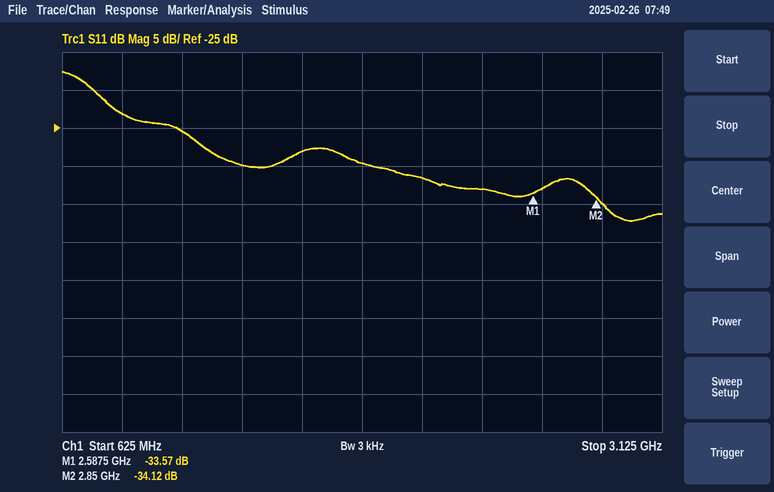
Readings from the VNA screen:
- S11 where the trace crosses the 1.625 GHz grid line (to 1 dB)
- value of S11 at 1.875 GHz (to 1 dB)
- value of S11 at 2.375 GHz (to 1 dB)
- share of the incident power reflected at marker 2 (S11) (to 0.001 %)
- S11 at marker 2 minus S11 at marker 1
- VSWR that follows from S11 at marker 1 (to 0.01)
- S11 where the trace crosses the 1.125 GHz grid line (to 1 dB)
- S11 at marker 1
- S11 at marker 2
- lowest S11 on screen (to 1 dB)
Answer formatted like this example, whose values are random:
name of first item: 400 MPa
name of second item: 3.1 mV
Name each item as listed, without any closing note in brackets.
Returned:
S11 where the trace crosses the 1.625 GHz grid line: -28 dB
value of S11 at 1.875 GHz: -30 dB
value of S11 at 2.375 GHz: -33 dB
share of the incident power reflected at marker 2 (S11): 0.039 %
S11 at marker 2 minus S11 at marker 1: -0.55 dB
VSWR that follows from S11 at marker 1: 1.04
S11 where the trace crosses the 1.125 GHz grid line: -25 dB
S11 at marker 1: -33.57 dB
S11 at marker 2: -34.12 dB
lowest S11 on screen: -37 dB
